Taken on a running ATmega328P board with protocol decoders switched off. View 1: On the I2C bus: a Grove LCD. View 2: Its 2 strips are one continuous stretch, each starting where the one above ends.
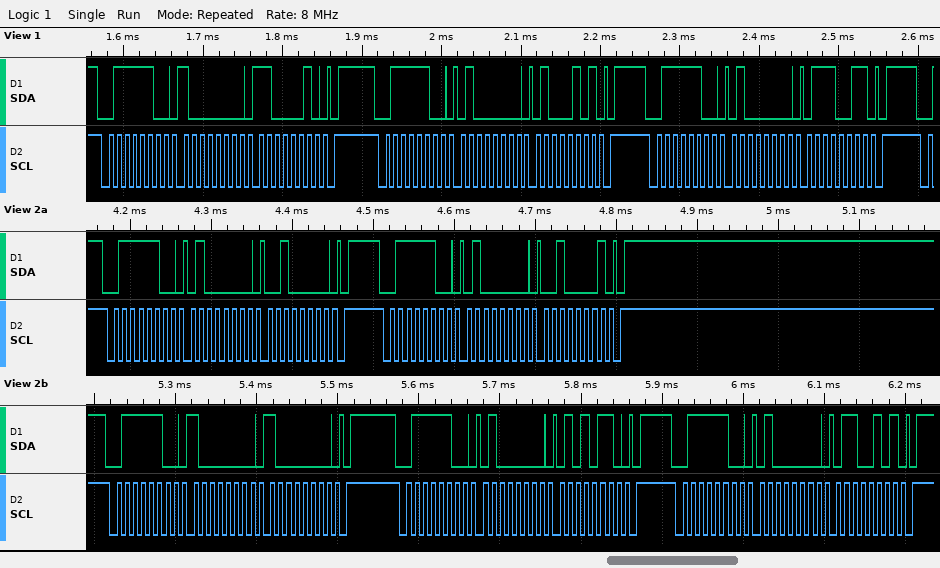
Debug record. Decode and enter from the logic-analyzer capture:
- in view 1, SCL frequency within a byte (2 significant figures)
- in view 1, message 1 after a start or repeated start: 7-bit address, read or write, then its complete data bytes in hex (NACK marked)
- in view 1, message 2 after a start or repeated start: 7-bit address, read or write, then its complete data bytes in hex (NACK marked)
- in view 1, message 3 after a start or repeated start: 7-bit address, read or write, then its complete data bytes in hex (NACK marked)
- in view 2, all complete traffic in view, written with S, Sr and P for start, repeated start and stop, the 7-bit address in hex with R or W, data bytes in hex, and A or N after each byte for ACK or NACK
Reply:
100 kHz
0x3E write: 80 C2
0x3E write: 40 45
0x3E write: 40 73
S 3EW A 40 A 20 A P S 3EW A 40 A 21 A P S 3EW A 80 A 80 A P S 3EW A 40 A 56 A P S 3EW A 40 A 65 A P
